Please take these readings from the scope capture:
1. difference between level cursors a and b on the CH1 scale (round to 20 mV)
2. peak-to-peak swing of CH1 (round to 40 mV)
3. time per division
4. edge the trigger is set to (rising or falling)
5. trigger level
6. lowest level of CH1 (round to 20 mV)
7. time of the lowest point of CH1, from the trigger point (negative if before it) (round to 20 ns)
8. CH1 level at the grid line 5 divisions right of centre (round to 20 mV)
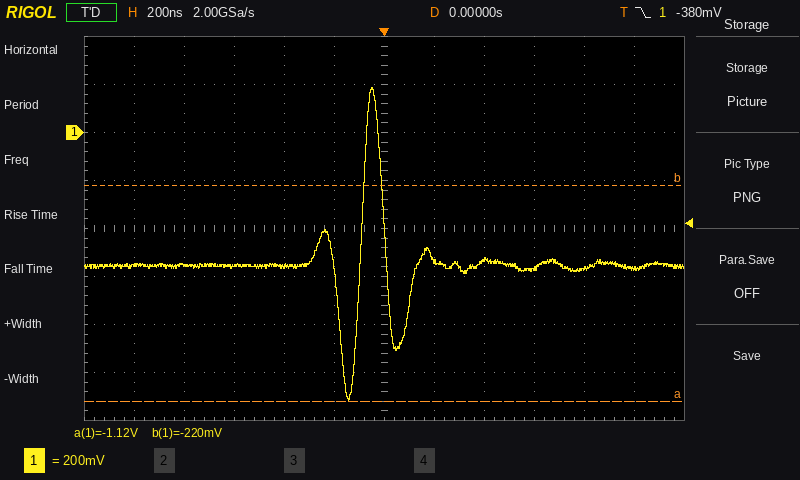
900 mV
1.32 V
200 ns
falling
-380 mV
-1.12 V
-140 ns
-560 mV
